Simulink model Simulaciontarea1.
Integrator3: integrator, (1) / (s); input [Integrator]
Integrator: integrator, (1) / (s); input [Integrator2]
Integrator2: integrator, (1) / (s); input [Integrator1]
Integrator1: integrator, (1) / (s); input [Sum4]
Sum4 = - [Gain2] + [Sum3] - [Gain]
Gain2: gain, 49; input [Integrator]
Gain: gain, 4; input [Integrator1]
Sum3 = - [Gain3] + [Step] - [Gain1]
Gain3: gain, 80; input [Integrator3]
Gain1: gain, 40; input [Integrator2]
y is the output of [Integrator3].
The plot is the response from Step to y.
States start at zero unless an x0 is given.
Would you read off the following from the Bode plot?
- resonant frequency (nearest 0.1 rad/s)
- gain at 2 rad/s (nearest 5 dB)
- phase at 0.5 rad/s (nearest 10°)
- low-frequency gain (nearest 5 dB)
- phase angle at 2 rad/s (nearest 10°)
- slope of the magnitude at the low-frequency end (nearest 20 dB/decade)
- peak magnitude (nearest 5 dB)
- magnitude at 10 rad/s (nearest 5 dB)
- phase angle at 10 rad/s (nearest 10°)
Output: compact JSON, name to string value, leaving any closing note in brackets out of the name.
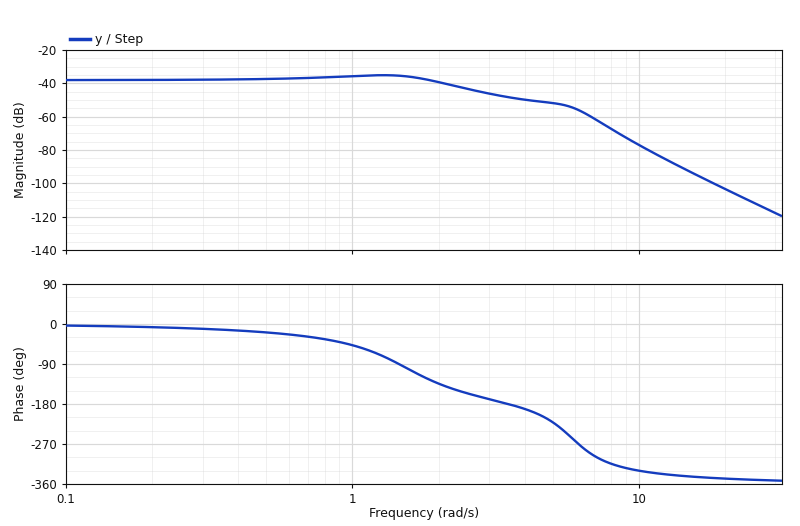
{"resonant frequency": "1.3 rad/s", "gain at 2 rad/s": "-40 dB", "phase at 0.5 rad/s": "-20°", "low-frequency gain": "-40 dB", "phase angle at 2 rad/s": "-130°", "slope of the magnitude at the low-frequency end": "0 dB/decade", "peak magnitude": "-35 dB", "magnitude at 10 rad/s": "-75 dB", "phase angle at 10 rad/s": "-330°"}
